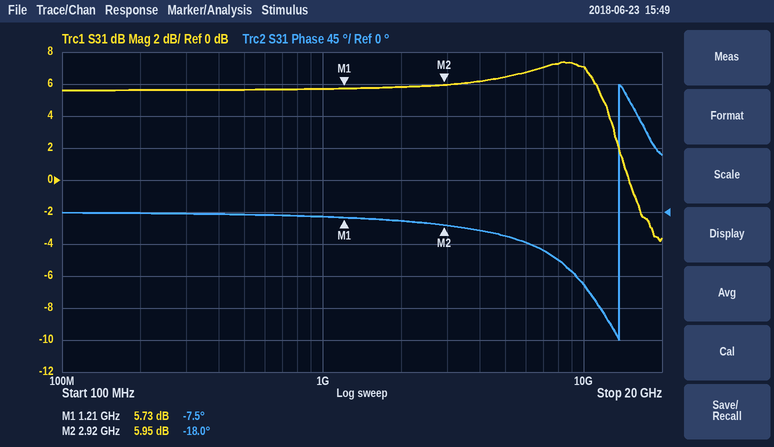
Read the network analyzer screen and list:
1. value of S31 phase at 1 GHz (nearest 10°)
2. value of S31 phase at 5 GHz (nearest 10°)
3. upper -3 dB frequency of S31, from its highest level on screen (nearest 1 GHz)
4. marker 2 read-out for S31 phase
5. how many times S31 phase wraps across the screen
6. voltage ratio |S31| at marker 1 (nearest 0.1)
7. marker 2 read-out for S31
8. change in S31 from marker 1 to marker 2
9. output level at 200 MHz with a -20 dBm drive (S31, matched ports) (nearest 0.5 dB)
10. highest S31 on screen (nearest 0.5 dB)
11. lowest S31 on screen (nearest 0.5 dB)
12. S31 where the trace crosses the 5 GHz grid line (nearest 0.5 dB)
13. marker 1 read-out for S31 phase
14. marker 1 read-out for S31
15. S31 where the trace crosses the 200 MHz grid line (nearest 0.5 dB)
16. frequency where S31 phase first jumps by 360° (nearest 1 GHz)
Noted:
-10°
-30°
12 GHz
-18.0°
1
1.9
5.95 dB
0.22 dB
-14.5 dBm
7.5 dB
-4.0 dB
6.5 dB
-7.5°
5.73 dB
5.5 dB
14 GHz
